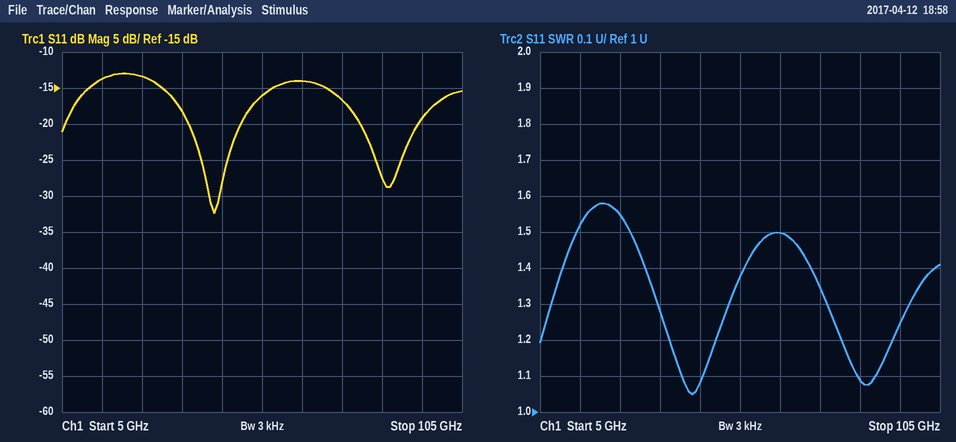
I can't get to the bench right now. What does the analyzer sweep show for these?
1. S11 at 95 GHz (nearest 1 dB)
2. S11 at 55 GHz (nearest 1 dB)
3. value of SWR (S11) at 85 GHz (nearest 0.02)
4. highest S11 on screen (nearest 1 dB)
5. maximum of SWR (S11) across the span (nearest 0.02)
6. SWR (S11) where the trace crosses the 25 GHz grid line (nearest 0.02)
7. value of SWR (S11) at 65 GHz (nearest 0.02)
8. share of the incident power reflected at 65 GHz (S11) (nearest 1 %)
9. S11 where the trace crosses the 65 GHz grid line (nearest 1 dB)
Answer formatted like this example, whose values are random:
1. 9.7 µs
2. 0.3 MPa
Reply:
1. -19 dB
2. -16 dB
3. 1.08
4. -13 dB
5. 1.58
6. 1.54
7. 1.50
8. 4 %
9. -14 dB
